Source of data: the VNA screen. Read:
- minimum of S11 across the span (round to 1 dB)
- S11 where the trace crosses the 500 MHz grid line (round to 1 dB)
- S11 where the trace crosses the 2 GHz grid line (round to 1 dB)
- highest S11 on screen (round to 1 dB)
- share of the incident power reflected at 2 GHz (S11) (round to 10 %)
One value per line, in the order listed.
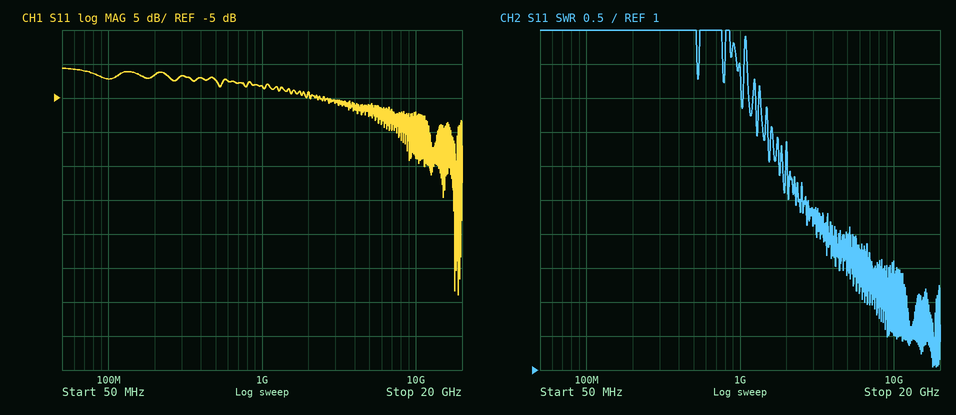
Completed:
-34 dB
-2 dB
-4 dB
-1 dB
40 %
